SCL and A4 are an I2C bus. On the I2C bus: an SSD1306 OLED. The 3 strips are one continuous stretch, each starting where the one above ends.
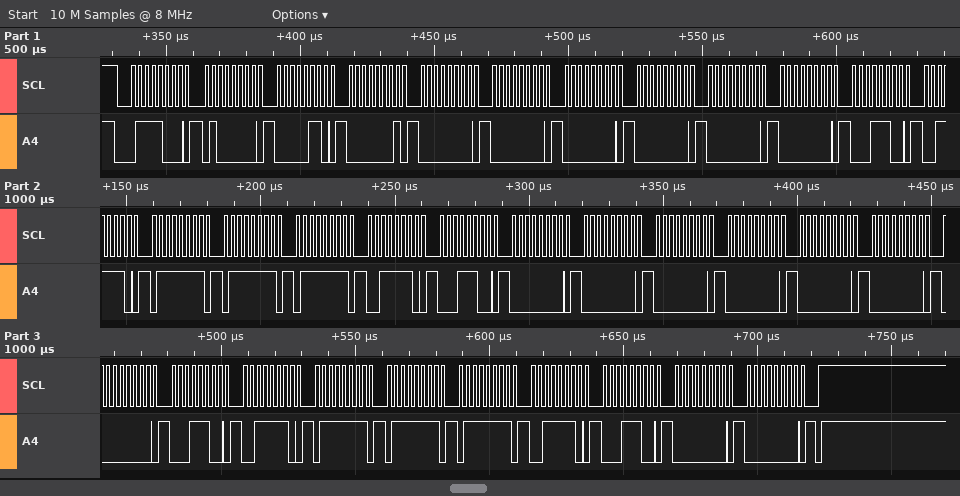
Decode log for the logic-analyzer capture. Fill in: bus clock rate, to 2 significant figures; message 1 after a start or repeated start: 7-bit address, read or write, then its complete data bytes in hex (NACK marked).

400 kHz
0x3C write: 40 06 01 00 00 00 00 00 00 1C 3E 7F 7F 7F 3E 1C 00 00 00 00 00 00 00 1C 3E 7F 7F 7F 3E 1C 00 00
